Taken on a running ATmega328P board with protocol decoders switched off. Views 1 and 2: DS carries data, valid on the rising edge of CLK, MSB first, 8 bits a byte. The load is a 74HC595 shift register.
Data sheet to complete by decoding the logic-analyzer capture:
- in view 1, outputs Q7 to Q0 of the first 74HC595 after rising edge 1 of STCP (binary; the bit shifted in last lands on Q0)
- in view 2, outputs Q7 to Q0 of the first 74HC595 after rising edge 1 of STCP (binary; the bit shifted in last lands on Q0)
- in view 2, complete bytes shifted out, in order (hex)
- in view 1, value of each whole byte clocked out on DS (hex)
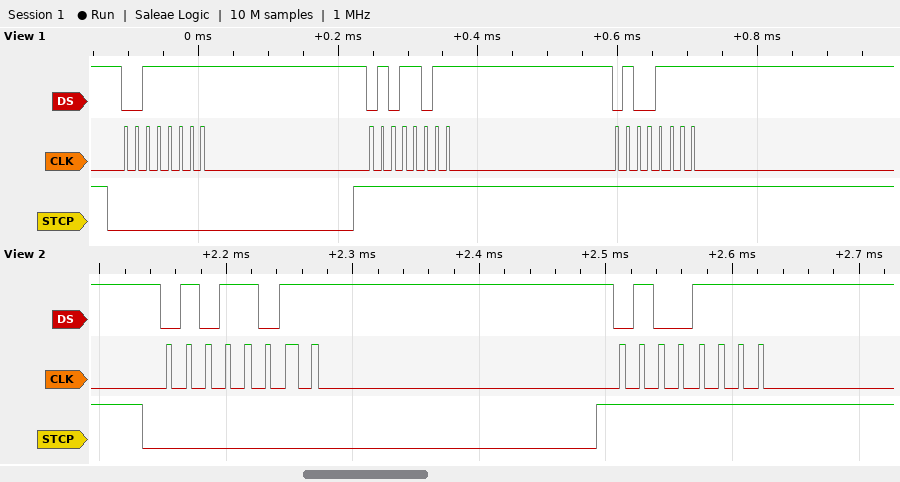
00111111
01011011
0x5B 0x4F
3F 5B 4F
